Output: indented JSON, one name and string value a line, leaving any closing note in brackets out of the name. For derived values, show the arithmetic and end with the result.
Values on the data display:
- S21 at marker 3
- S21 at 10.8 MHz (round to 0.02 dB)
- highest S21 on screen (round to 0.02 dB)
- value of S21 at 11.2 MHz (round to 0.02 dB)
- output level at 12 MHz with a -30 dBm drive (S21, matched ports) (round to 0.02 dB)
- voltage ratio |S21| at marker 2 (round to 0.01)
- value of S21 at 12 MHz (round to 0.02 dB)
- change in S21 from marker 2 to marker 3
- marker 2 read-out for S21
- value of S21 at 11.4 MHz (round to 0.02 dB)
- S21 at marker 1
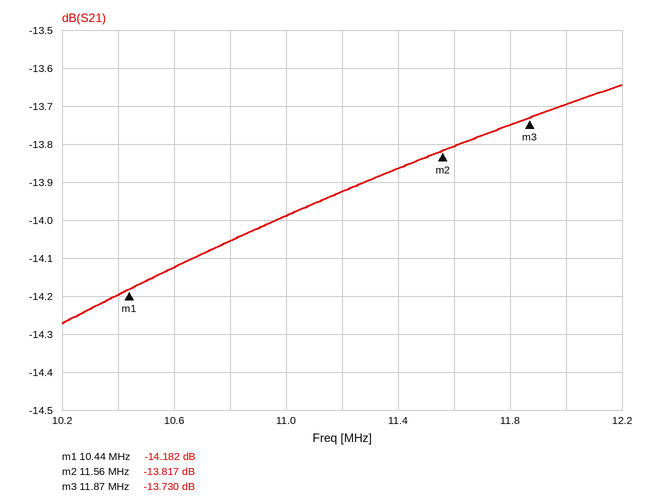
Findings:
{
  "S21 at marker 3": "-13.730 dB",
  "S21 at 10.8 MHz": "-14.06 dB",
  "highest S21 on screen": "-13.64 dB",
  "value of S21 at 11.2 MHz": "-13.92 dB",
  "output level at 12 MHz with a -30 dBm drive (S21, matched ports)": "-30 dBm + (-13.70 dB) = -43.70 dBm",
  "voltage ratio |S21| at marker 2": "10^(-13.817/20) ≈ 0.20",
  "value of S21 at 12 MHz": "-13.70 dB",
  "change in S21 from marker 2 to marker 3": "-13.73 − (-13.817) = 0.087 dB",
  "marker 2 read-out for S21": "-13.817 dB",
  "value of S21 at 11.4 MHz": "-13.86 dB",
  "S21 at marker 1": "-14.182 dB"
}
